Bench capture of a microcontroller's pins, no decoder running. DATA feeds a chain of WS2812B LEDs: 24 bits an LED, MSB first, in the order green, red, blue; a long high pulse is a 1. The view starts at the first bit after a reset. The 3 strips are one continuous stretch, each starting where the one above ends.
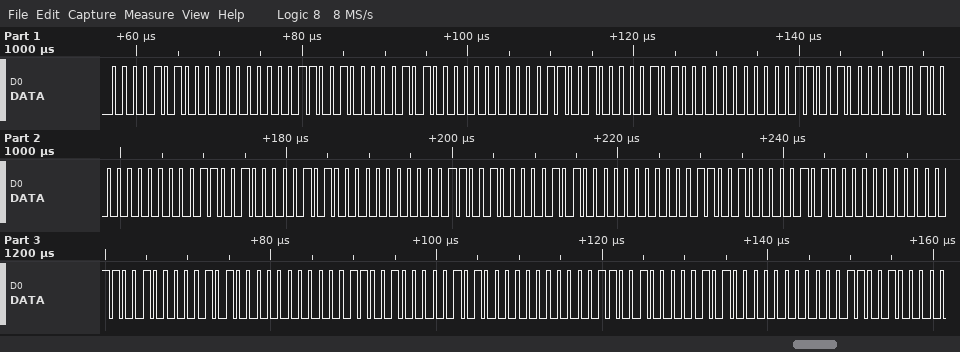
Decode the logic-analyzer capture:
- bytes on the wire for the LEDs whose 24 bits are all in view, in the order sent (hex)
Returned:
0A 00 32 0A 00 32 0A 00 32 0A 00 32 0A 00 32 0A 00 32 0A 00 32 0A 00 32 0A 00 32 0A 00 32
